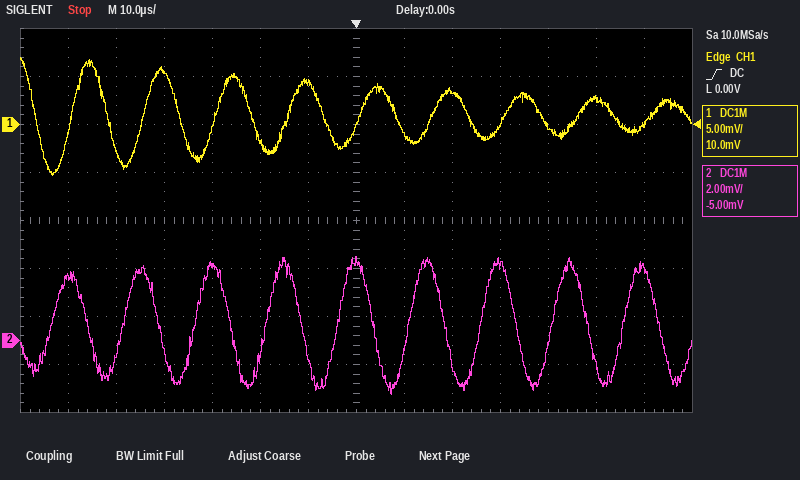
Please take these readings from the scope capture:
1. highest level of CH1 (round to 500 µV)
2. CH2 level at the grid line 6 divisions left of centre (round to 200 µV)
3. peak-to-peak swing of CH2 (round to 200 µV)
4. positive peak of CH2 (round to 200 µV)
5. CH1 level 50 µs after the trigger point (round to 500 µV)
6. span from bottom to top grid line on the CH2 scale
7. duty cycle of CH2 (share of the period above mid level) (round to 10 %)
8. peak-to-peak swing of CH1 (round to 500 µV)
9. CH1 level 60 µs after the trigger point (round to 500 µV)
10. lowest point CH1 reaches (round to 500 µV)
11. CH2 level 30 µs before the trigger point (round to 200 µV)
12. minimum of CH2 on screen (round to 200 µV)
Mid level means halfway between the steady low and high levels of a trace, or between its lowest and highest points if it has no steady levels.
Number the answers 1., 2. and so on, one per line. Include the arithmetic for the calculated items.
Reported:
1. 7.0 mV
2. 2.6 mV
3. 3.6 mV − (-2.2 mV) = 5.8 mV
4. 3.6 mV
5. 2.5 mV
6. 16 mV
7. 50 %
8. 7.0 mV − (-5.5 mV) = 12.5 mV
9. 0.0 mV
10. -5.5 mV
11. 3.2 mV
12. -2.2 mV
